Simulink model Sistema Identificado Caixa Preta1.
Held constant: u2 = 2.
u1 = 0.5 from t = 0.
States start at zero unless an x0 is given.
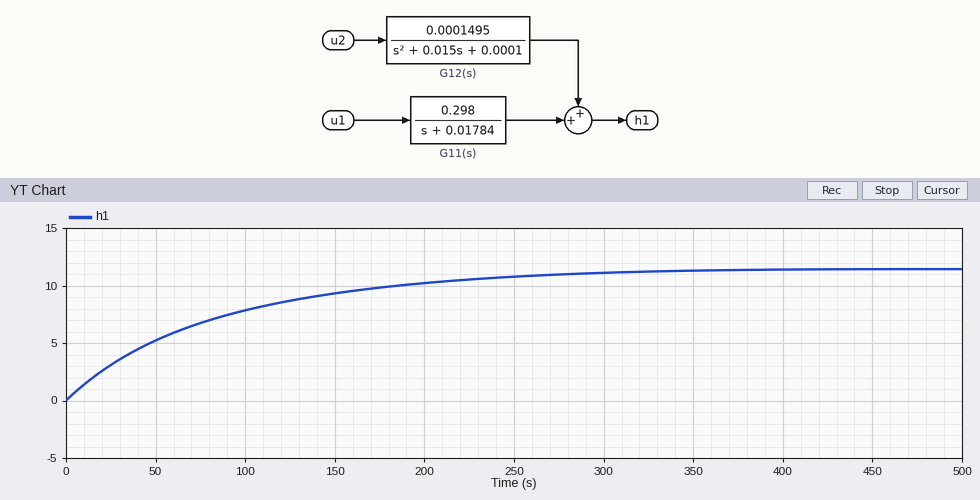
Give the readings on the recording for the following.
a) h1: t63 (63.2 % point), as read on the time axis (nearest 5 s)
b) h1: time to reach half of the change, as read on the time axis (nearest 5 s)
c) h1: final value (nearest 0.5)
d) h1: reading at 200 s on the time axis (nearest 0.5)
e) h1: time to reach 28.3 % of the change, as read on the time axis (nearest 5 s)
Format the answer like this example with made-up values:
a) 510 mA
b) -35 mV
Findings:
a) 85 s
b) 55 s
c) 11.5
d) 10.0
e) 25 s
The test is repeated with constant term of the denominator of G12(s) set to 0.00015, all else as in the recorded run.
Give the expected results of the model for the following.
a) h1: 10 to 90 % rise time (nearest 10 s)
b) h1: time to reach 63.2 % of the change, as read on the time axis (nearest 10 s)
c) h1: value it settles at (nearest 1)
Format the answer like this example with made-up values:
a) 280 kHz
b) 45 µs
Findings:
a) 150 s
b) 70 s
c) 10
